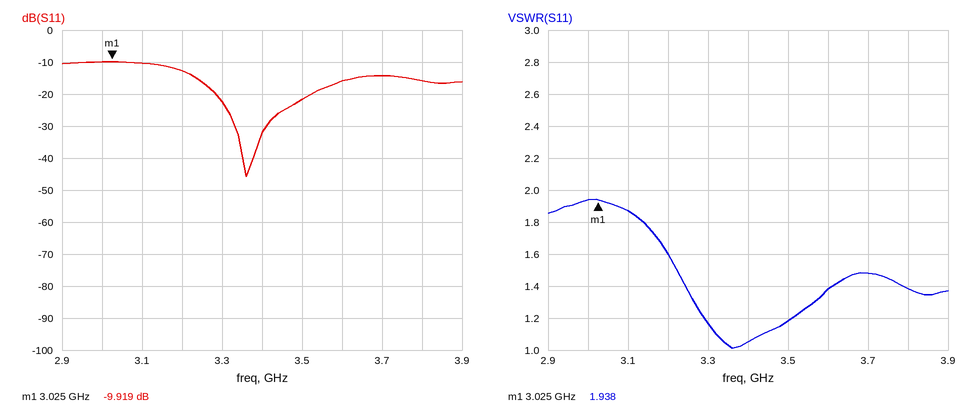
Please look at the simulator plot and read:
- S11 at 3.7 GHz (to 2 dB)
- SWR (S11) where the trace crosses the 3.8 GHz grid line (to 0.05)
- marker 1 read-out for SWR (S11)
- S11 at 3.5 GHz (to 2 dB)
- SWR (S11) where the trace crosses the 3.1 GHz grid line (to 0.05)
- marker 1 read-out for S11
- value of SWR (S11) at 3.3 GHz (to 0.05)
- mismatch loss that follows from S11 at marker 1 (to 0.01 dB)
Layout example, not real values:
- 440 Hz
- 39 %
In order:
- -14 dB
- 1.40
- 1.938
- -22 dB
- 1.85
- -9.919 dB
- 1.15
- 0.47 dB
